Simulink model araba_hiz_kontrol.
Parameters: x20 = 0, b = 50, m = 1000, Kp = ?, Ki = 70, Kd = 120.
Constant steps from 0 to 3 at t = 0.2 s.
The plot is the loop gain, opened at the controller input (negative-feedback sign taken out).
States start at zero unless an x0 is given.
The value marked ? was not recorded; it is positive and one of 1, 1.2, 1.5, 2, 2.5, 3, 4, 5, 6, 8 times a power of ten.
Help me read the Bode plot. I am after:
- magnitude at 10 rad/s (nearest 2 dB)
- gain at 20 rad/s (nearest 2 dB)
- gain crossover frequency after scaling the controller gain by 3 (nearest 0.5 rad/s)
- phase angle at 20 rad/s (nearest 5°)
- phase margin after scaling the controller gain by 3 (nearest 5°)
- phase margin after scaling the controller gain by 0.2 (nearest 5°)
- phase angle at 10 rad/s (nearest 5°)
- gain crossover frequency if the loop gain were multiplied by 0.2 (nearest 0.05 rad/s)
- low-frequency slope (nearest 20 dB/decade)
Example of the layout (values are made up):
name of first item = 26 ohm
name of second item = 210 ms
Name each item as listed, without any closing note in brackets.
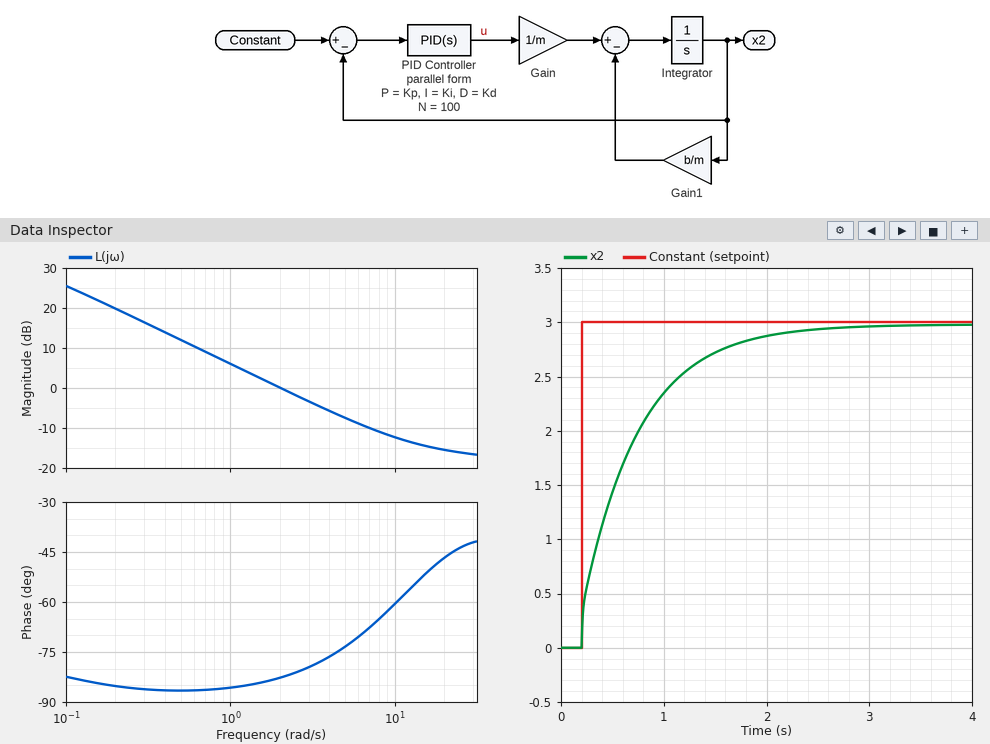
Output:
magnitude at 10 rad/s = -12 dB
gain at 20 rad/s = -16 dB
gain crossover frequency after scaling the controller gain by 3 = 6.5 rad/s
phase angle at 20 rad/s = -45°
phase margin after scaling the controller gain by 3 = 110°
phase margin after scaling the controller gain by 0.2 = 95°
phase angle at 10 rad/s = -60°
gain crossover frequency if the loop gain were multiplied by 0.2 = 0.40 rad/s
low-frequency slope = -20 dB/decade
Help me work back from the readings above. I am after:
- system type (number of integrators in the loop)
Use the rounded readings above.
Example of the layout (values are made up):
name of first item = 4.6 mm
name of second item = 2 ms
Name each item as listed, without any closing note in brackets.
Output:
system type = 1
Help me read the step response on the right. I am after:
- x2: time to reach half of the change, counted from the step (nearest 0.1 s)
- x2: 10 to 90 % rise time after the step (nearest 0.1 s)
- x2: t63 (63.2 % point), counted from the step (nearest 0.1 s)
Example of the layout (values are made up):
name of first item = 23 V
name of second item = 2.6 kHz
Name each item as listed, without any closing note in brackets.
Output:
x2: time to reach half of the change, counted from the step = 0.3 s
x2: 10 to 90 % rise time after the step = 1.2 s
x2: t63 (63.2 % point), counted from the step = 0.5 s
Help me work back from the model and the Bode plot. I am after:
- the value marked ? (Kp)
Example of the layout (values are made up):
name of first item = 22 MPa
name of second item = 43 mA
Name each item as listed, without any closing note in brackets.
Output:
the value marked ? = 2000
